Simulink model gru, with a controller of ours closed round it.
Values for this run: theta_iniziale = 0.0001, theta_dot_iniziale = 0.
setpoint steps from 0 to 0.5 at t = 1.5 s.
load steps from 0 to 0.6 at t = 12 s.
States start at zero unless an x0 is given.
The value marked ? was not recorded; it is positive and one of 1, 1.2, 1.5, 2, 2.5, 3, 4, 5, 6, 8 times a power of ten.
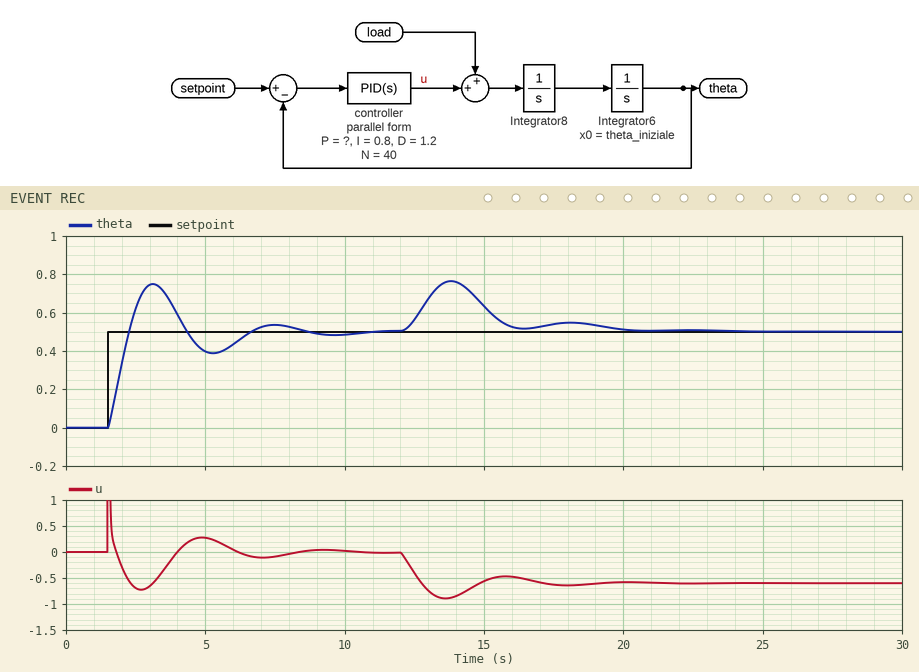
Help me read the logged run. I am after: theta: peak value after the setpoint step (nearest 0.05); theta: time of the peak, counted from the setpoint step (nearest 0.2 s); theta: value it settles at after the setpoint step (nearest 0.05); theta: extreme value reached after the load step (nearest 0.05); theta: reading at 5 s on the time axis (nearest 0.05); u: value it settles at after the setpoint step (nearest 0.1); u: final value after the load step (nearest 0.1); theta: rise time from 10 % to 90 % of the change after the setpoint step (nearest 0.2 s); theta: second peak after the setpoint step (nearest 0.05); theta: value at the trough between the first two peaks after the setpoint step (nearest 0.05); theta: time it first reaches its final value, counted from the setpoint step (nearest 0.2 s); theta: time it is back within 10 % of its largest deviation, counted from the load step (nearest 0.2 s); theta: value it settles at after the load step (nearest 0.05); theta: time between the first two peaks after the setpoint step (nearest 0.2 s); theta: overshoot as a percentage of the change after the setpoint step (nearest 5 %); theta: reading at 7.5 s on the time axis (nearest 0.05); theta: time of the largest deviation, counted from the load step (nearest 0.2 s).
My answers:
0.75
1.6 s
0.50
0.75
0.40
0.0
-0.6
0.6 s
0.55
0.40
0.8 s
7.4 s
0.50
4.4 s
50 %
0.55
1.8 s
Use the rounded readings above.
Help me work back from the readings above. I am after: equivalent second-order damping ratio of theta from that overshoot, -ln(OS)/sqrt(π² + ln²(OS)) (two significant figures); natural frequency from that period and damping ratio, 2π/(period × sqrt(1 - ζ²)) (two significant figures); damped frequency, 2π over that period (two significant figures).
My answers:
0.22
1.5 rad/s
1.4 rad/s
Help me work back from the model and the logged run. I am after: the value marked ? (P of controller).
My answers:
2.5
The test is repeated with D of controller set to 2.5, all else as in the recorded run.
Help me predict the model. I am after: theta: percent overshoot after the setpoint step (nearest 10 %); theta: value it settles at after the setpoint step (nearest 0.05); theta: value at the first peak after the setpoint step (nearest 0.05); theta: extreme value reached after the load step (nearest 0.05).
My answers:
20 %
0.50
0.60
0.70
